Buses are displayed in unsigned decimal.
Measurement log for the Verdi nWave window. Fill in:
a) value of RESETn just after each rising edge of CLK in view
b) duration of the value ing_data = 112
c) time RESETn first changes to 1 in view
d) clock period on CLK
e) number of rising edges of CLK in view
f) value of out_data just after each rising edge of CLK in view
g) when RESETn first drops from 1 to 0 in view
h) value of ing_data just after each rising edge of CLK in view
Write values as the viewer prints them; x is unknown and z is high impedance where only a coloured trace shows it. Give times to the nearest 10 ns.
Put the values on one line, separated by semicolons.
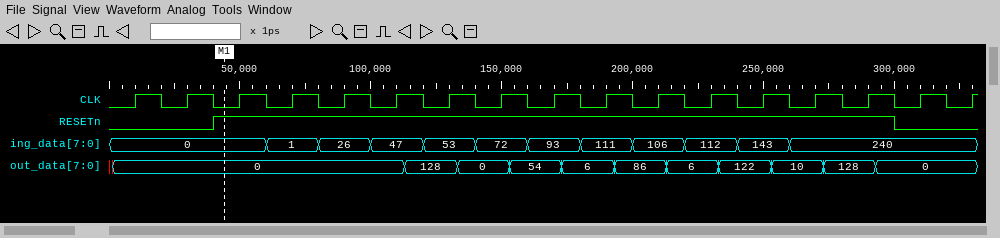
0 0 1 1 1 1 1 1 1 1 1 1 1 1 1 0 0; 20 ns; 40 ns; 20 ns; 17; 0, 0, 0, 0, 0, 0, 128, 0, 54, 6, 86, 6, 122, 10, 128, 0, 0; 300 ns; 0, 0, 0, 1, 26, 47, 53, 72, 93, 111, 106, 112, 143, 240, 240, 240, 240
